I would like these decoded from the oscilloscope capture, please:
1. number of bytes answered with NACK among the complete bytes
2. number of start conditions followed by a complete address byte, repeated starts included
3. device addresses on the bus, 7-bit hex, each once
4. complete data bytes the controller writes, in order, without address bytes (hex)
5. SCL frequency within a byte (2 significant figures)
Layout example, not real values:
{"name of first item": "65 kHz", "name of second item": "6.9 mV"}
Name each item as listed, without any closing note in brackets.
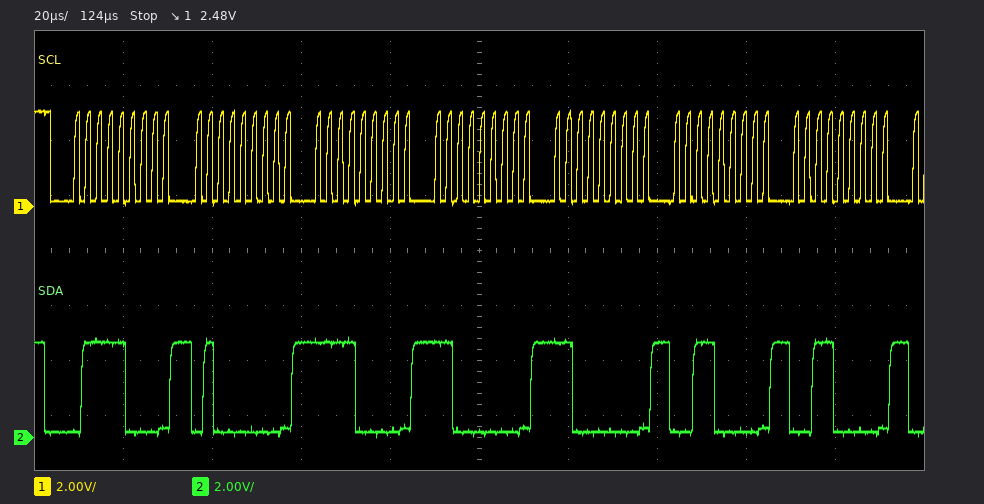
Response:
{"number of bytes answered with NACK among the complete bytes": "0", "number of start conditions followed by a complete address byte, repeated starts included": "1", "device addresses on the bus, 7-bit hex, each once": "0x3C", "complete data bytes the controller writes, in order, without address bytes": "40 F0 C0 C0 30 30", "SCL frequency within a byte": "400 kHz"}
